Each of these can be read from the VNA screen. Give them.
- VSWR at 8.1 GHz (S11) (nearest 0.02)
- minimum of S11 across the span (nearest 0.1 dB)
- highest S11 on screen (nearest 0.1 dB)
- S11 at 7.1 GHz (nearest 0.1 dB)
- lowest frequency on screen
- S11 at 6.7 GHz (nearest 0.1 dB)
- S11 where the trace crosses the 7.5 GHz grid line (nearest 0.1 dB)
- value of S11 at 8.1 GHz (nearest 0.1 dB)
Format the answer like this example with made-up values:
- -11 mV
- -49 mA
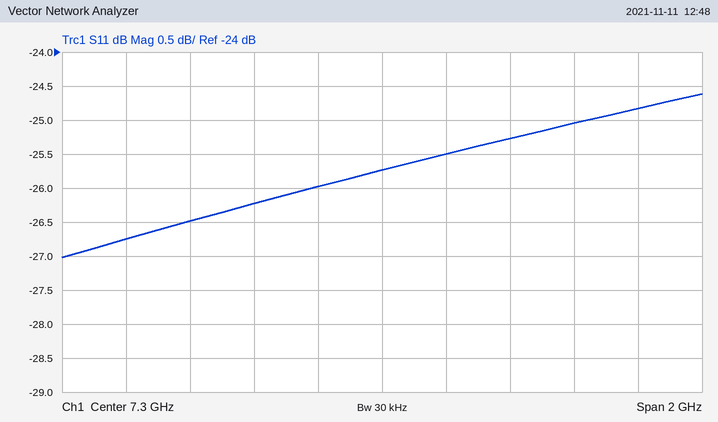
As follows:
- 1.12
- -27.0 dB
- -24.6 dB
- -26.0 dB
- 6.3 GHz
- -26.5 dB
- -25.5 dB
- -24.8 dB
